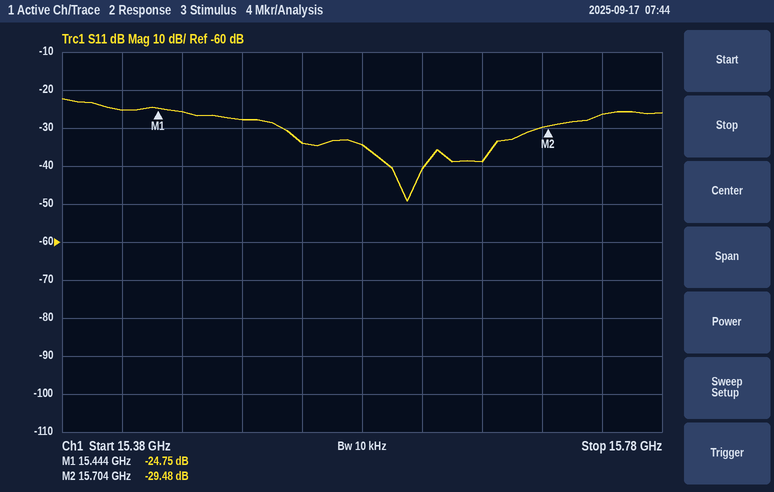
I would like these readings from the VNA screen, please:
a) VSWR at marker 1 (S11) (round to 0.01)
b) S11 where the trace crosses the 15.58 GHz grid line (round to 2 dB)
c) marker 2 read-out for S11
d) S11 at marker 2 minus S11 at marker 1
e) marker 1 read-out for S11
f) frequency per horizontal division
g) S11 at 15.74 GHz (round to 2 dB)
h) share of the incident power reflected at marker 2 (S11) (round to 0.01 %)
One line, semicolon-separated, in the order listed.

1.12; -34 dB; -29.48 dB; -4.73 dB; -24.75 dB; 40 MHz; -26 dB; 0.11 %
